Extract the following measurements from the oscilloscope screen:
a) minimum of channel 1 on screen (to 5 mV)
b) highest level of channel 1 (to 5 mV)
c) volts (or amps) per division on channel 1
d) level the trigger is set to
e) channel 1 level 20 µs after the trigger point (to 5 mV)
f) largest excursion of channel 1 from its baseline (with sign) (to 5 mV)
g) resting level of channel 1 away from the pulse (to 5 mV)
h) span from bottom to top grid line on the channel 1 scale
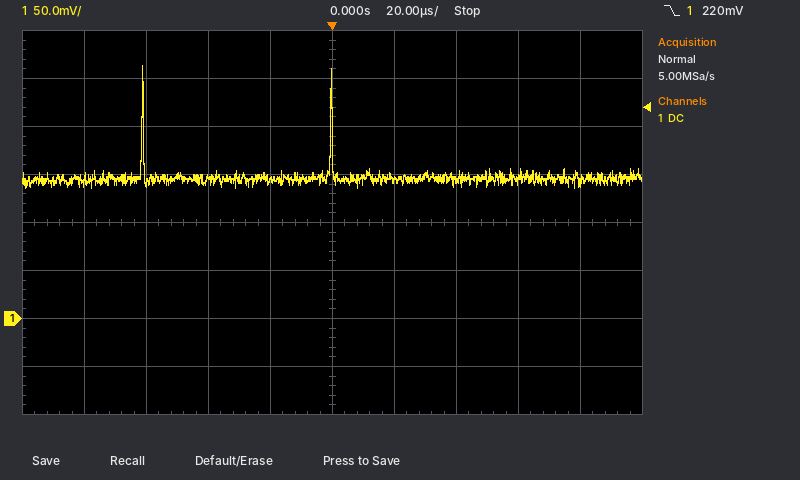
135 mV
265 mV
50 mV
220 mV
145 mV
+120 mV
145 mV
400 mV
